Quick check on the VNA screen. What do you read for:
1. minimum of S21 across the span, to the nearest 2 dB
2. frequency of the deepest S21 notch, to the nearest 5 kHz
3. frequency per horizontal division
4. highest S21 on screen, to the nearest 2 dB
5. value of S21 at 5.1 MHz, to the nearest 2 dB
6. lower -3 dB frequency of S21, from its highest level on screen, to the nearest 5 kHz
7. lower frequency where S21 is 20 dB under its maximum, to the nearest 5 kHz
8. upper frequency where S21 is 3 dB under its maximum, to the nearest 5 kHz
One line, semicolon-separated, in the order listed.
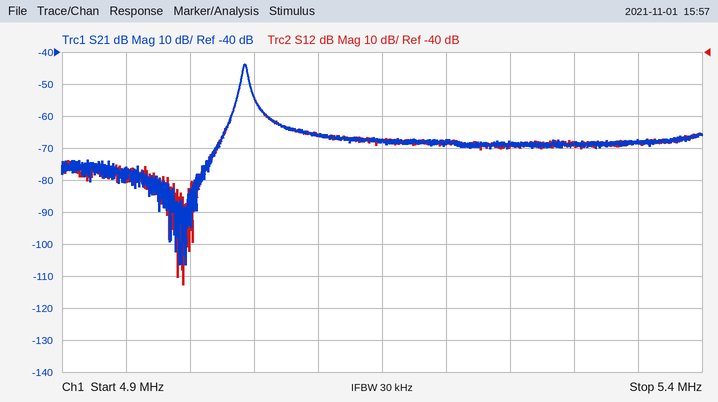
-106 dB; 4.990 MHz; 50 kHz; -44 dB; -66 dB; 5.040 MHz; 5.030 MHz; 5.045 MHz
